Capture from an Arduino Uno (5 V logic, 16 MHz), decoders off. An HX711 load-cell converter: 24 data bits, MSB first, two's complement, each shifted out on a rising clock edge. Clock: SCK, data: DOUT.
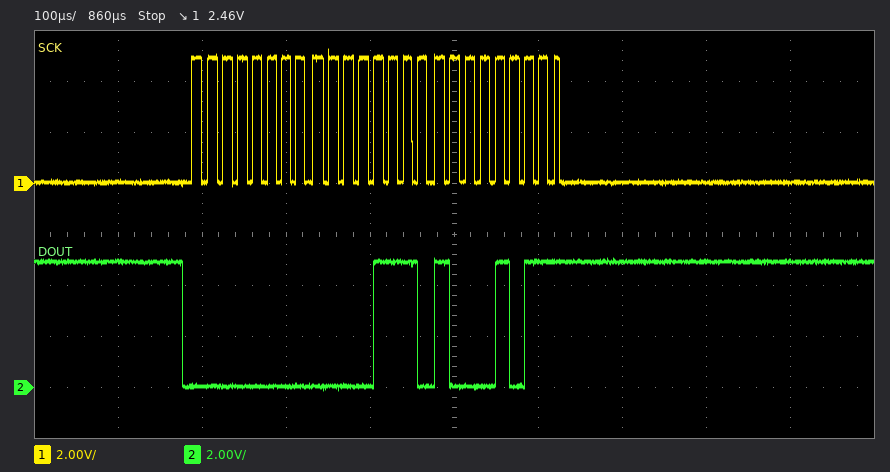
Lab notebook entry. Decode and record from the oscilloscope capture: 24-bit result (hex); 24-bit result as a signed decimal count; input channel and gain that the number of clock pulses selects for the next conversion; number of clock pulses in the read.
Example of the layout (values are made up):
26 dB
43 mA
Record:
0x000E8B
3723
channel A, gain 128
25
